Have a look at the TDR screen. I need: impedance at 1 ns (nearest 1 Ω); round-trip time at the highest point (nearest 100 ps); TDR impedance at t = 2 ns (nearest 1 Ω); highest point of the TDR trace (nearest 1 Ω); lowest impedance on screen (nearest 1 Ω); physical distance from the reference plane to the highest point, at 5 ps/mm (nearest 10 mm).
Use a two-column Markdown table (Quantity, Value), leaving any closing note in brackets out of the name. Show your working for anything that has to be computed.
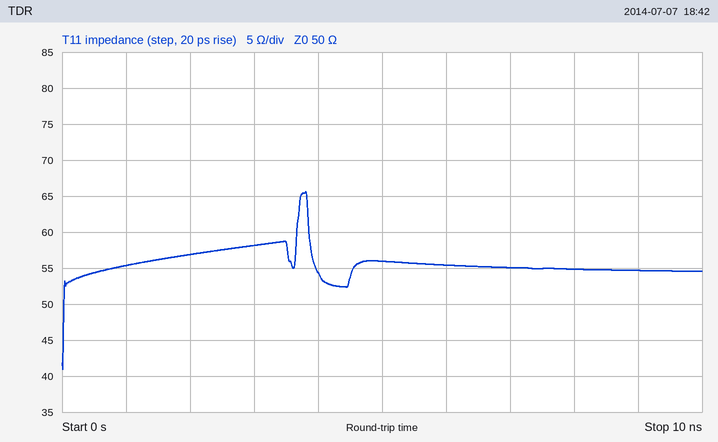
| Quantity | Value |
|---|---|
| impedance at 1 ns | 55 Ω |
| round-trip time at the highest point | 3.8 ns |
| TDR impedance at t = 2 ns | 57 Ω |
| highest point of the TDR trace | 66 Ω |
| lowest impedance on screen | 41 Ω |
| physical distance from the reference plane to the highest point, at 5 ps/mm | 3.8 ns / 2 / 5 ps/mm ≈ 380 mm |
